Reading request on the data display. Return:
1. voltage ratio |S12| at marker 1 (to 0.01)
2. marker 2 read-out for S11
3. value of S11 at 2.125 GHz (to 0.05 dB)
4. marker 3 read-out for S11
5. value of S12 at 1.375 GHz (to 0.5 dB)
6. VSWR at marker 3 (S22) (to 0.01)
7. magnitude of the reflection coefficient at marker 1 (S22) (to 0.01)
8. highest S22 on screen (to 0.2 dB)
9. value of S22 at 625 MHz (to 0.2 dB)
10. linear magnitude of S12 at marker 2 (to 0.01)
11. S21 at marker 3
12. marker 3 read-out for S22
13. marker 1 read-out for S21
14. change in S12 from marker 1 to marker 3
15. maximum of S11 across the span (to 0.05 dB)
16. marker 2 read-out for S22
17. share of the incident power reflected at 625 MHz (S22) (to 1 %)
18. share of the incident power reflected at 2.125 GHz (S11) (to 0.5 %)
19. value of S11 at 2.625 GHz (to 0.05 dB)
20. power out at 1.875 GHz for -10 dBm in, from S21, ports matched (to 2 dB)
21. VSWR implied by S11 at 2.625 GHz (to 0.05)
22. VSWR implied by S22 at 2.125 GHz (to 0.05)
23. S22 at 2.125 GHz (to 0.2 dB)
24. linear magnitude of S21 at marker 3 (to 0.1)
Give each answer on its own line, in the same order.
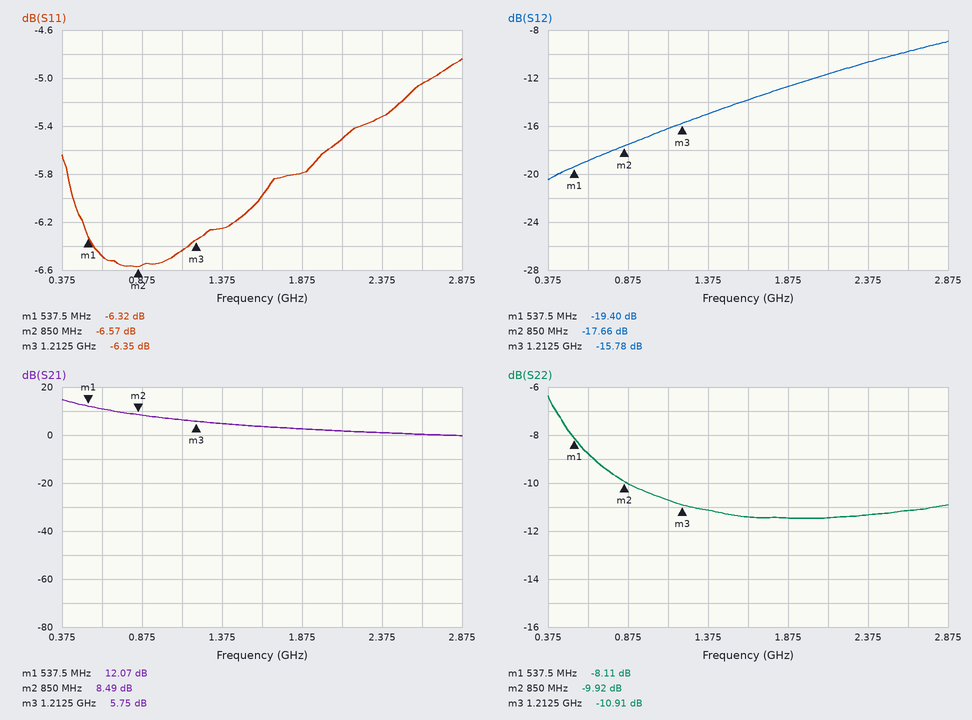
0.11
-6.57 dB
-5.50 dB
-6.35 dB
-15.0 dB
1.80
0.39
-6.4 dB
-8.8 dB
0.13
5.75 dB
-10.91 dB
12.07 dB
3.62 dB
-4.85 dB
-9.92 dB
13 %
28.0 %
-5.05 dB
-8 dBm
3.55
1.75
-11.4 dB
1.9
